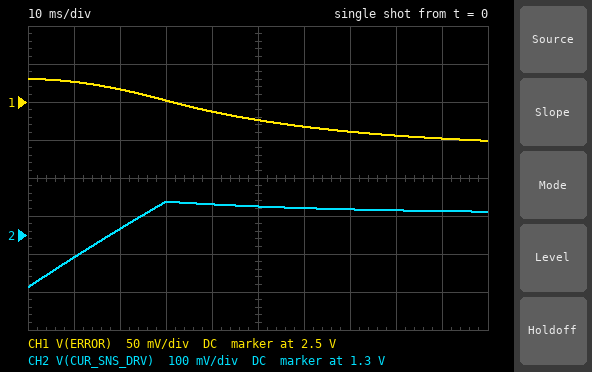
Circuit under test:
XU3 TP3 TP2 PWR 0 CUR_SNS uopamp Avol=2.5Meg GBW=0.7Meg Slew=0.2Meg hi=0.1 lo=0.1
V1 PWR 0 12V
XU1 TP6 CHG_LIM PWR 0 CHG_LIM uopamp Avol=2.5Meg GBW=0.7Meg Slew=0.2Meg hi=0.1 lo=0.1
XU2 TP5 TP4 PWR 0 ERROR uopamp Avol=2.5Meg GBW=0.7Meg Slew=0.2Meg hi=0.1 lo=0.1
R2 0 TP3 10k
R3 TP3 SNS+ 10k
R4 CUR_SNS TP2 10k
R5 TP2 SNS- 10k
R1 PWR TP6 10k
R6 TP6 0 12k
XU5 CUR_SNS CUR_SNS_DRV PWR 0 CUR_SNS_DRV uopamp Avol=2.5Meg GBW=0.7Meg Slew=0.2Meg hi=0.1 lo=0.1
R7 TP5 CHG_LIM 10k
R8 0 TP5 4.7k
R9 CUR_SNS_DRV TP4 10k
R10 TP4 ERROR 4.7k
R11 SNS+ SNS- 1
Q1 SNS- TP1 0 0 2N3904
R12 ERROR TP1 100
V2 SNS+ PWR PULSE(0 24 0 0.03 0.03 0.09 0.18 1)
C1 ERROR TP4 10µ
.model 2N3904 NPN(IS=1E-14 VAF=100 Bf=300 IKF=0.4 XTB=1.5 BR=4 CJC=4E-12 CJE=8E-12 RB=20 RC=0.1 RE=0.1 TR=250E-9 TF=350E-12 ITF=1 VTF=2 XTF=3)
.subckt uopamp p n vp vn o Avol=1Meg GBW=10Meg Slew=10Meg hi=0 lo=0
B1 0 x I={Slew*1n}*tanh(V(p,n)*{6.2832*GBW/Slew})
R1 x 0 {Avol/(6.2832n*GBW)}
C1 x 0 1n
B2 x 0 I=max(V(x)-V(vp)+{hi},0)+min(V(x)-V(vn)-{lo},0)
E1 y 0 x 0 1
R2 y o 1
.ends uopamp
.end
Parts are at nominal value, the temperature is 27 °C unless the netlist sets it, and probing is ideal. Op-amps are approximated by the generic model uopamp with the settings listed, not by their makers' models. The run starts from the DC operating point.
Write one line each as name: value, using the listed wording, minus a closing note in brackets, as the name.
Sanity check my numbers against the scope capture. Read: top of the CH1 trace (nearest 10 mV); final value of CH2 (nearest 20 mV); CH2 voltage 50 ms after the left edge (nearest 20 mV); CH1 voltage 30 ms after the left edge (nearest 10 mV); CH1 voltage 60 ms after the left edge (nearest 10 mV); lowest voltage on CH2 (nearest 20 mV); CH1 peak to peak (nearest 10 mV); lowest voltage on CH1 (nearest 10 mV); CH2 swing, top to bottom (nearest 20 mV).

top of the CH1 trace: 2.53 V
final value of CH2: 1.36 V
CH2 voltage 50 ms after the left edge: 1.38 V
CH1 voltage 30 ms after the left edge: 2.50 V
CH1 voltage 60 ms after the left edge: 2.47 V
lowest voltage on CH2: 1.16 V
CH1 peak to peak: 80 mV
lowest voltage on CH1: 2.45 V
CH2 swing, top to bottom: 220 mV
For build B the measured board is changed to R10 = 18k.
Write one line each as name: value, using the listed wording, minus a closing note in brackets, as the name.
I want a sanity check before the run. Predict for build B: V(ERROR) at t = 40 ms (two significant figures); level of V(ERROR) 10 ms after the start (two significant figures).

V(ERROR) at t = 40 ms: 3.2 V
level of V(ERROR) 10 ms after the start: 3.3 V
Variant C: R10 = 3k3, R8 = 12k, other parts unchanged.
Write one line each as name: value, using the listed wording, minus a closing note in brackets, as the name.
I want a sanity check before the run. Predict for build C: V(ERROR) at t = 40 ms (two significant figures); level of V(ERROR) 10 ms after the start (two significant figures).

V(ERROR) at t = 40 ms: 4.1 V
level of V(ERROR) 10 ms after the start: 4.2 V
